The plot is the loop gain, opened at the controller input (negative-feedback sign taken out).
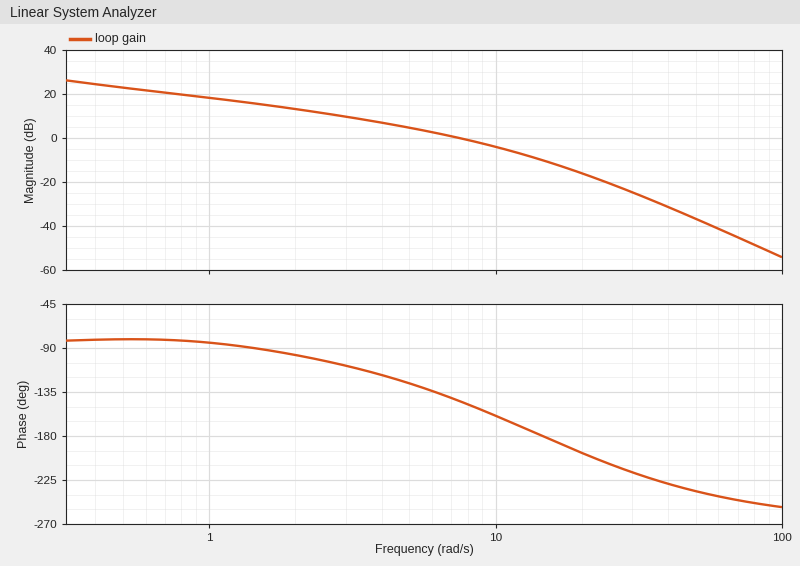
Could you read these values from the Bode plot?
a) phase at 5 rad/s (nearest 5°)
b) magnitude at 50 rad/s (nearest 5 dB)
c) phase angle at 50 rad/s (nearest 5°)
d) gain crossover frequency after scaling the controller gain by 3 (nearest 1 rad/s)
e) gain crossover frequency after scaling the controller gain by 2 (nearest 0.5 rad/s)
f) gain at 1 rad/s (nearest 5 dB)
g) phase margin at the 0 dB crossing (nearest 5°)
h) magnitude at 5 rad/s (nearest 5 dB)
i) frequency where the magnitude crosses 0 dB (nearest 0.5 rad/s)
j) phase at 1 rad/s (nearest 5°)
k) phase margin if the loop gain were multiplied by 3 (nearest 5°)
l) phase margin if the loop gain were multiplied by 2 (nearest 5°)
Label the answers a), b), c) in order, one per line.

a) -125°
b) -35 dB
c) -235°
d) 14 rad/s
e) 11.5 rad/s
f) 20 dB
g) 35°
h) 5 dB
i) 7.5 rad/s
j) -85°
k) 0°
l) 15°
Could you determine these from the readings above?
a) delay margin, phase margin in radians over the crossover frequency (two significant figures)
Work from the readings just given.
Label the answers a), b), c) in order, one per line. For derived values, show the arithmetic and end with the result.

a) 35 × π / 180 / 7.5 = 0.081 s
